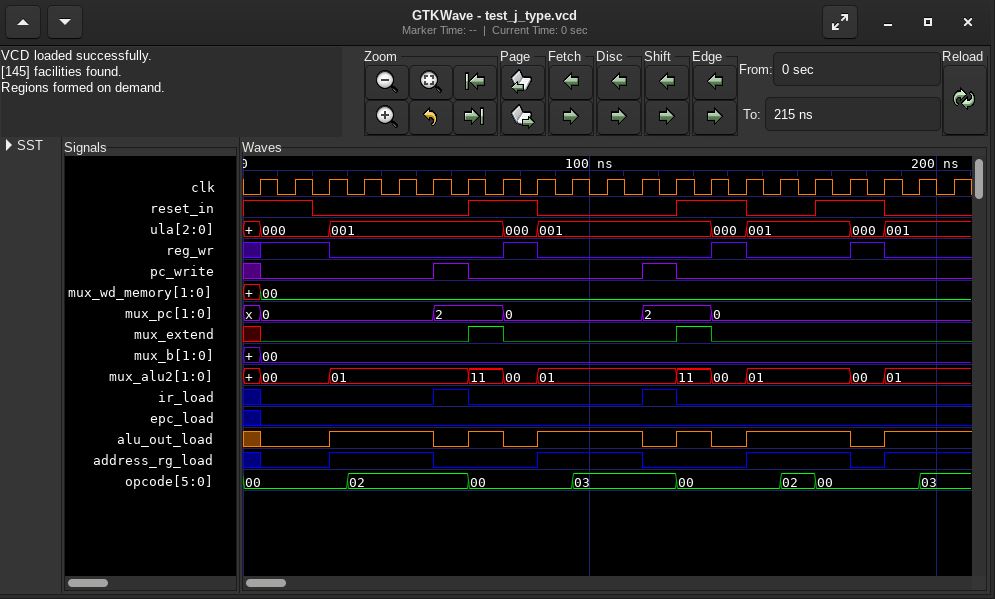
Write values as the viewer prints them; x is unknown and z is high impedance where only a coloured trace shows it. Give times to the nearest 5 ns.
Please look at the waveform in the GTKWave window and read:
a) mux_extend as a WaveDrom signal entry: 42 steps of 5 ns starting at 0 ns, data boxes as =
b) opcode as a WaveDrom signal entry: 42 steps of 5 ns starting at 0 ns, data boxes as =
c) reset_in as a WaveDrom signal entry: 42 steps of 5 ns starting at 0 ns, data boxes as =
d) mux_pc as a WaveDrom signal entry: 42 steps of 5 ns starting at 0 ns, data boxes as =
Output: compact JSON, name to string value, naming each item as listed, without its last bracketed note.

{"mux_extend as a WaveDrom signal entry: 42 steps of 5 ns starting at 0 ns, data boxes as =": "{name: 'mux_extend', wave: 'x0...........1.0.........1.0..............'}", "opcode as a WaveDrom signal entry: 42 steps of 5 ns starting at 0 ns, data boxes as =": "{name: 'opcode', wave: '=.....=......=.....=.....=.....=.=.....=..', data: '00 02 00 03 00 02 00 03'}", "reset_in as a WaveDrom signal entry: 42 steps of 5 ns starting at 0 ns, data boxes as =": "{name: 'reset_in', wave: '1...0........1...0.......1...0...1...0....'}", "mux_pc as a WaveDrom signal entry: 42 steps of 5 ns starting at 0 ns, data boxes as =": "{name: 'mux_pc', wave: 'x=.........=...=.......=...=..............', data: '0 2 0 2 0'}"}
